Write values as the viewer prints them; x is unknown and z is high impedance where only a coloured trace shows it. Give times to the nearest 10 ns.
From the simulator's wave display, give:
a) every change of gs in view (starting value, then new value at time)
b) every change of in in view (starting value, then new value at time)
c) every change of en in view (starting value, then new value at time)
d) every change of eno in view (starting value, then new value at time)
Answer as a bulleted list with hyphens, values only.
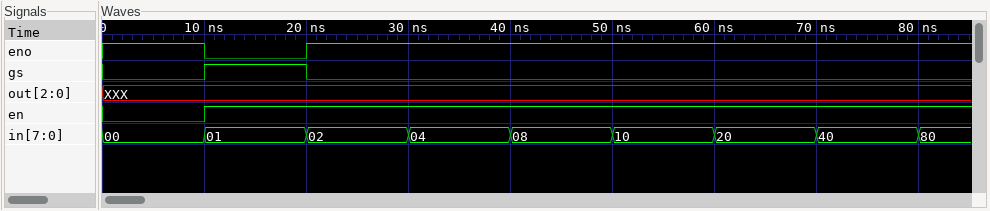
- 0, 1 at 10 ns, 0 at 20 ns
- 00, 01 at 10 ns, 02 at 20 ns, 04 at 30 ns, 08 at 40 ns, 10 at 50 ns, 20 at 60 ns, 40 at 70 ns, 80 at 80 ns
- 0, 1 at 10 ns
- 1, 0 at 10 ns, 1 at 20 ns
